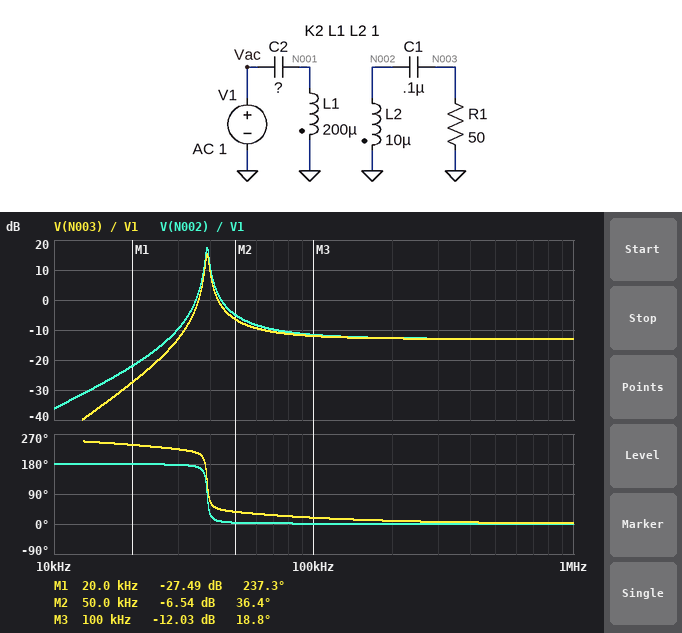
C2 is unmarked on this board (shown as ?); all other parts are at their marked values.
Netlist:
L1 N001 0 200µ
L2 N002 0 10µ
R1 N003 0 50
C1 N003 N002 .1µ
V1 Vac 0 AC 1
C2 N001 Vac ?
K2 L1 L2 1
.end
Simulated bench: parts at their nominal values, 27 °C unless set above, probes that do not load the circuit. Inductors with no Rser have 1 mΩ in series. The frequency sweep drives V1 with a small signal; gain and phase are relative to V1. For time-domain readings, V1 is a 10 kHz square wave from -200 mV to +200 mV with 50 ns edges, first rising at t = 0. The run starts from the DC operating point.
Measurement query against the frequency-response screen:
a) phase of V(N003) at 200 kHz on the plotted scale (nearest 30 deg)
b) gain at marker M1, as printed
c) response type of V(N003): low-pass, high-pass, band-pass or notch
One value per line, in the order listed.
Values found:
0 deg
-27.49 dB
high-pass
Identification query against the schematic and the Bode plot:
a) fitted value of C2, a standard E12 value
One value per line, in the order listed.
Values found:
82 nF
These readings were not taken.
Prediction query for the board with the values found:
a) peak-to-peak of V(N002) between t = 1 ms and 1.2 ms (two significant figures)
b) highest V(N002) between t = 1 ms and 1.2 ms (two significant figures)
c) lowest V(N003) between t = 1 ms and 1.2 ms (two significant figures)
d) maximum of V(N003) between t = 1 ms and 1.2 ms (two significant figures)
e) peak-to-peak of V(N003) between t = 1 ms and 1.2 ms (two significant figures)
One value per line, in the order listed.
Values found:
99 mV
49 mV
-61 mV
62 mV
120 mV
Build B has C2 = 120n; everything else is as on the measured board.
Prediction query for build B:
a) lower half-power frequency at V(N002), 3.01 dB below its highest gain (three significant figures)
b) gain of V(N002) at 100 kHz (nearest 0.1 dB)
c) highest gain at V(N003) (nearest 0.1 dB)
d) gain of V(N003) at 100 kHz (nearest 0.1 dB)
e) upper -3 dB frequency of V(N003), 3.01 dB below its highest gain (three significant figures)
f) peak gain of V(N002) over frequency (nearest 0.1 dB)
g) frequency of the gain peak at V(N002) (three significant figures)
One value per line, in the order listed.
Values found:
31.8 kHz
-12.1 dB
17.6 dB
-12.5 dB
32.5 kHz
20.6 dB
32.2 kHz
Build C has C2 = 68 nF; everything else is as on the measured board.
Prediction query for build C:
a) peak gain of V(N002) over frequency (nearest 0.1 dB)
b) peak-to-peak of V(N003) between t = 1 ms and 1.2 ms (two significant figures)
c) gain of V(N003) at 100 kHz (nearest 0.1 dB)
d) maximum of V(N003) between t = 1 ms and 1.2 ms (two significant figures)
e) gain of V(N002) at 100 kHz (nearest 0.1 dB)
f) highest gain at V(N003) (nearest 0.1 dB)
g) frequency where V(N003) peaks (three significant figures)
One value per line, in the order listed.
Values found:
16.0 dB
150 mV
-11.7 dB
75 mV
-11.3 dB
14.1 dB
42.6 kHz
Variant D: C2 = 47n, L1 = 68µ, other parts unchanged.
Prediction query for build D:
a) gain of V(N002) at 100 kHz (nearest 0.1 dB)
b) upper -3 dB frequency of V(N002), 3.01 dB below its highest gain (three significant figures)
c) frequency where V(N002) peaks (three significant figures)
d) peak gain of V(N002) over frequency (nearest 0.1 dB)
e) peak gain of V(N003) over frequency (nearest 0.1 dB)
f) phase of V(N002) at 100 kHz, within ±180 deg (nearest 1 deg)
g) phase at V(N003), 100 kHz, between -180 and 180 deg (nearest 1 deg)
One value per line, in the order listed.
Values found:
3.6 dB
92.4 kHz
87.6 kHz
11.6 dB
11.1 dB
21 deg
39 deg
